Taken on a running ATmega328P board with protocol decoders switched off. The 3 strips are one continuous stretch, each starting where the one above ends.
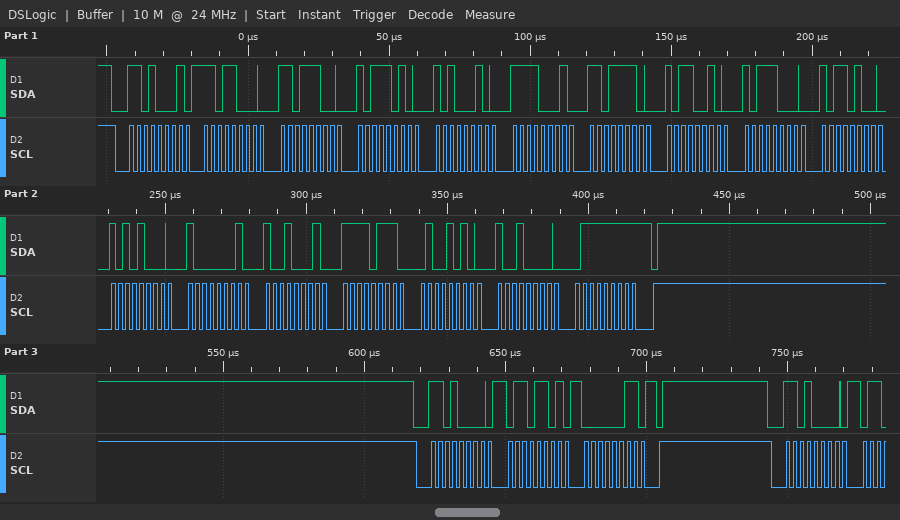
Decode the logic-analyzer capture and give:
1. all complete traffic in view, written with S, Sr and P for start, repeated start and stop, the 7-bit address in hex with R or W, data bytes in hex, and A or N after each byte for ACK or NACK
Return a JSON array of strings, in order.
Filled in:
["S 68R A D8 A DC A BA A A2 A F1 A DE A B2 A B8 A B4 A A8 A 81 A 91 A F7 A 4A A 90 A 7F N P S 68W A 6D A 03 A P S 68W A"]
